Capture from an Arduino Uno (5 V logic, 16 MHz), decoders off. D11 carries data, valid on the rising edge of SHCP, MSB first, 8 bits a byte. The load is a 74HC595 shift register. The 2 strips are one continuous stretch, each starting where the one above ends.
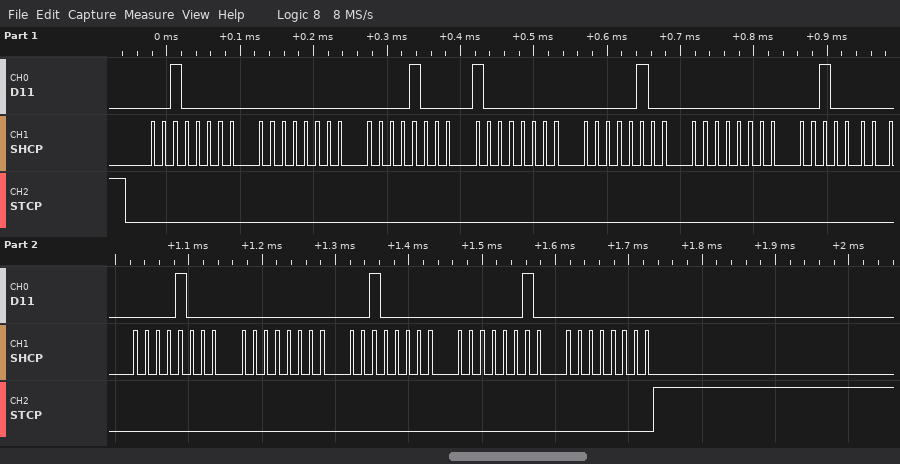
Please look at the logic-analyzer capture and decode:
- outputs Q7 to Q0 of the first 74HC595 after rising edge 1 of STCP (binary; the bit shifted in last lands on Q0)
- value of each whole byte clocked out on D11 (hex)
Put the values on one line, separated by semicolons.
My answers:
00000000; 20 00 08 80 04 00 20 08 00 20 02 00
